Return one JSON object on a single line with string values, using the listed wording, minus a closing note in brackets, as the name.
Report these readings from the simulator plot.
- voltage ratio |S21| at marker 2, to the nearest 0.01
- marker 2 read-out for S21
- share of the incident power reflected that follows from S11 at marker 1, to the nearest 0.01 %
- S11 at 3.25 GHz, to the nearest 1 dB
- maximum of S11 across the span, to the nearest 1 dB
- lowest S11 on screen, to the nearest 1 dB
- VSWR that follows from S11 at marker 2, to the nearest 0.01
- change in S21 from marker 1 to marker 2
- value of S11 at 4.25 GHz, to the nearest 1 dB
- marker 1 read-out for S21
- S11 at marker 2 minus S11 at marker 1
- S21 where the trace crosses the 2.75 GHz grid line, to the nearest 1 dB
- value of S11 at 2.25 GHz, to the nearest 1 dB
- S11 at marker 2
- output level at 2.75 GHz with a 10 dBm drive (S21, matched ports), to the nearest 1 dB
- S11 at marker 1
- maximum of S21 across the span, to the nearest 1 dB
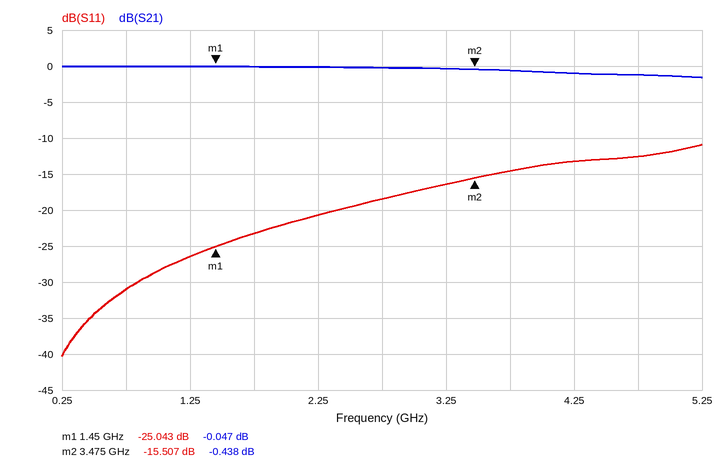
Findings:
{"voltage ratio |S21| at marker 2, to the nearest 0.01": "0.95", "marker 2 read-out for S21": "-0.438 dB", "share of the incident power reflected that follows from S11 at marker 1, to the nearest 0.01 %": "0.31 %", "S11 at 3.25 GHz, to the nearest 1 dB": "-16 dB", "maximum of S11 across the span, to the nearest 1 dB": "-11 dB", "lowest S11 on screen, to the nearest 1 dB": "-40 dB", "VSWR that follows from S11 at marker 2, to the nearest 0.01": "1.40", "change in S21 from marker 1 to marker 2": "-0.391 dB", "value of S11 at 4.25 GHz, to the nearest 1 dB": "-13 dB", "marker 1 read-out for S21": "-0.047 dB", "S11 at marker 2 minus S11 at marker 1": "9.536 dB", "S21 where the trace crosses the 2.75 GHz grid line, to the nearest 1 dB": "0 dB", "value of S11 at 2.25 GHz, to the nearest 1 dB": "-21 dB", "S11 at marker 2": "-15.507 dB", "output level at 2.75 GHz with a 10 dBm drive (S21, matched ports), to the nearest 1 dB": "10 dBm", "S11 at marker 1": "-25.043 dB", "maximum of S21 across the span, to the nearest 1 dB": "0 dB"}
